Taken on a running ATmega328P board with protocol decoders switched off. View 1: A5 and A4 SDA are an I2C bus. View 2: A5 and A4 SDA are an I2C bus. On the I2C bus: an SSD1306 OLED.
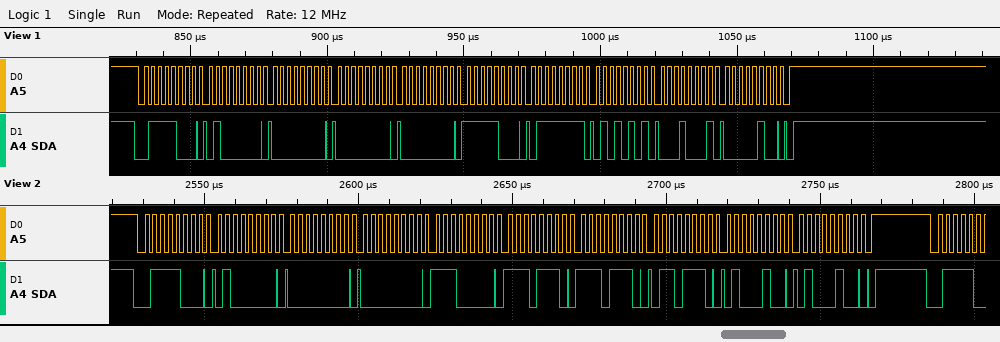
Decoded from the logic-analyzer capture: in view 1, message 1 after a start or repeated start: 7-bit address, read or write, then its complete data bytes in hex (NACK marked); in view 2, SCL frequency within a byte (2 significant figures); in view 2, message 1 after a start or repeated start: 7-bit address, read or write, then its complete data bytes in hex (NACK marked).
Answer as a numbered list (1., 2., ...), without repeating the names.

1. 0x3C write: 40 00 00 00 F8 7F 55 11 04
2. 400 kHz
3. 0x3C write: 40 00 00 E0 EE EE 6E 44 44
